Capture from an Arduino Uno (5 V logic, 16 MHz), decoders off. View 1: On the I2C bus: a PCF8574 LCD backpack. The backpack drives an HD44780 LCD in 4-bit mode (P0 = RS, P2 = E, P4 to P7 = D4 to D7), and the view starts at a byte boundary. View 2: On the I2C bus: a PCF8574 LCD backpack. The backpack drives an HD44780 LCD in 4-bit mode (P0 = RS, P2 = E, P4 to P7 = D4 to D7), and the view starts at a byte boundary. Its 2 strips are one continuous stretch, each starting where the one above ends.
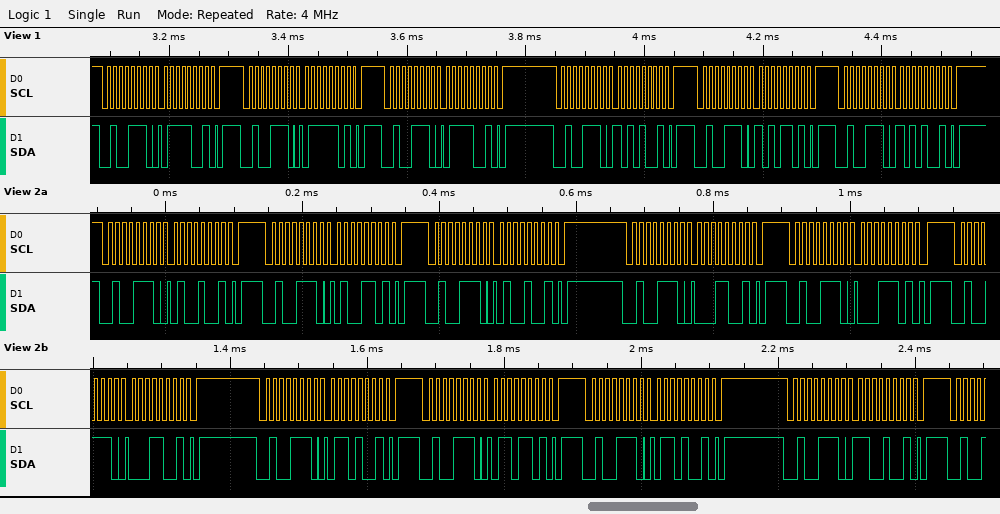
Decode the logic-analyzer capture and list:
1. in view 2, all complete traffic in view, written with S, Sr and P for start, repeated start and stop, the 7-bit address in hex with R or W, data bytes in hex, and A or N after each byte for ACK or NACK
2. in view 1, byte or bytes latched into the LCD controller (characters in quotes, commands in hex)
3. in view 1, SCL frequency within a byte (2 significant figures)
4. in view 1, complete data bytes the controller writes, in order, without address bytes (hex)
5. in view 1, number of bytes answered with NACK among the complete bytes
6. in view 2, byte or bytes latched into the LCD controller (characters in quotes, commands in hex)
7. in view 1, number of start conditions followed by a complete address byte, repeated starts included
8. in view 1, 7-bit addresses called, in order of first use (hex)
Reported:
S 27W A 49 A P S 27W A 4D A P S 27W A 49 A P S 27W A 19 A P S 27W A 1D A P S 27W A 19 A P S 27W A 69 A P S 27W A 6D A P S 27W A 69 A P S 27W A C9 A P
'z'
100 kHz
79 7D 79 A9 AD A9
0
'A'
6
0x27
